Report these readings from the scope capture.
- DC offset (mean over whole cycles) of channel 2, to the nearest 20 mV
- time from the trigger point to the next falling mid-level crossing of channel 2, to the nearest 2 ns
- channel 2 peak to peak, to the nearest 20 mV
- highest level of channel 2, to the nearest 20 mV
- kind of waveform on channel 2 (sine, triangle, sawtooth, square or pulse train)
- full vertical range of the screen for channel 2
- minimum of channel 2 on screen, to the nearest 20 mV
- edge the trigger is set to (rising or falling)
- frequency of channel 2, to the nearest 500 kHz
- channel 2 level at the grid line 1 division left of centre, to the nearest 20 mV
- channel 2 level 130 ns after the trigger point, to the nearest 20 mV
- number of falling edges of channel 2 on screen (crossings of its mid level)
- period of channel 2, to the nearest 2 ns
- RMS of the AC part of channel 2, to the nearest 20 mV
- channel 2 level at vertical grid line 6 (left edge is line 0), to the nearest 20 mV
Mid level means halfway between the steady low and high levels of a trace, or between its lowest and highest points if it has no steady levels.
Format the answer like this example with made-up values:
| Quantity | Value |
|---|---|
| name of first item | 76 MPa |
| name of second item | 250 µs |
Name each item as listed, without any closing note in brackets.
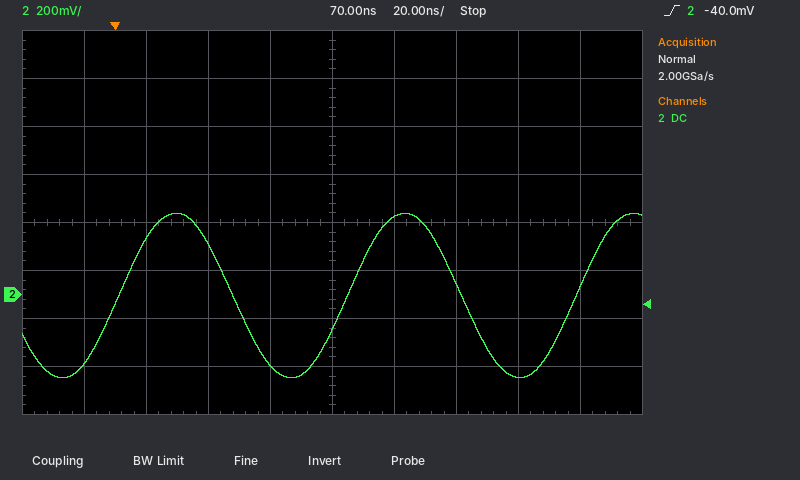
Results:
| Quantity | Value |
|---|---|
| DC offset (mean over whole cycles) of channel 2, to the nearest 20 mV | 0 mV |
| time from the trigger point to the next falling mid-level crossing of channel 2, to the nearest 2 ns | 38 ns |
| channel 2 peak to peak, to the nearest 20 mV | 680 mV |
| highest level of channel 2, to the nearest 20 mV | 340 mV |
| kind of waveform on channel 2 | sine |
| full vertical range of the screen for channel 2 | 1.6 V |
| minimum of channel 2 on screen, to the nearest 20 mV | -340 mV |
| edge the trigger is set to | rising |
| frequency of channel 2, to the nearest 500 kHz | 13.5 MHz |
| channel 2 level at the grid line 1 division left of centre, to the nearest 20 mV | -300 mV |
| channel 2 level 130 ns after the trigger point, to the nearest 20 mV | -340 mV |
| number of falling edges of channel 2 on screen | 2 |
| period of channel 2, to the nearest 2 ns | 74 ns |
| RMS of the AC part of channel 2, to the nearest 20 mV | 240 mV |
| channel 2 level at vertical grid line 6 (left edge is line 0), to the nearest 20 mV | 320 mV |
